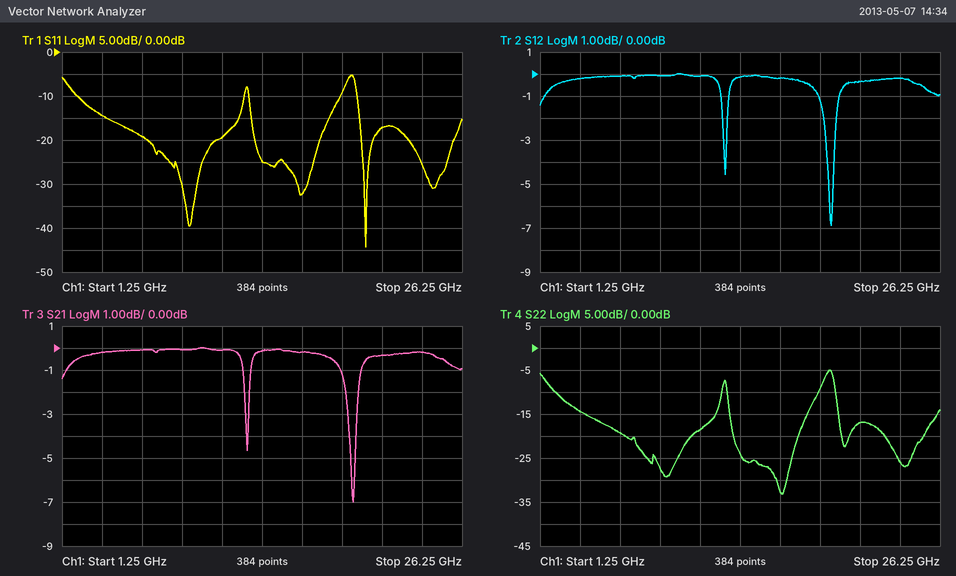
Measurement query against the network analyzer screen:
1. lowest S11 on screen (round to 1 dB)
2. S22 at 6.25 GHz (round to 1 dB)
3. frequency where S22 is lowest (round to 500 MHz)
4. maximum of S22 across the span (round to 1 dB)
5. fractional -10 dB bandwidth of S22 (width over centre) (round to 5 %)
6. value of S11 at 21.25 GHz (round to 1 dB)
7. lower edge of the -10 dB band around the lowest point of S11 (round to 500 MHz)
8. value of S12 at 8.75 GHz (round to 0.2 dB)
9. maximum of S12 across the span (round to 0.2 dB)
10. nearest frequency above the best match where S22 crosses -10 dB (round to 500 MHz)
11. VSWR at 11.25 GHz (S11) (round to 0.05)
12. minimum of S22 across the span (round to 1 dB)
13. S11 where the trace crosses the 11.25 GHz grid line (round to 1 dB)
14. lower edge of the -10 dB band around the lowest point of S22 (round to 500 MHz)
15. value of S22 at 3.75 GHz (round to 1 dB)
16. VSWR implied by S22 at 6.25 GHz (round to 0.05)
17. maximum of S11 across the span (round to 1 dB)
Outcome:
-44 dB
-19 dB
16.5 GHz
-5 dB
35 %
-17 dB
19.5 GHz
0.0 dB
0.0 dB
18.5 GHz
1.25
-33 dB
-19 dB
13.0 GHz
-14 dB
1.25
-5 dB
